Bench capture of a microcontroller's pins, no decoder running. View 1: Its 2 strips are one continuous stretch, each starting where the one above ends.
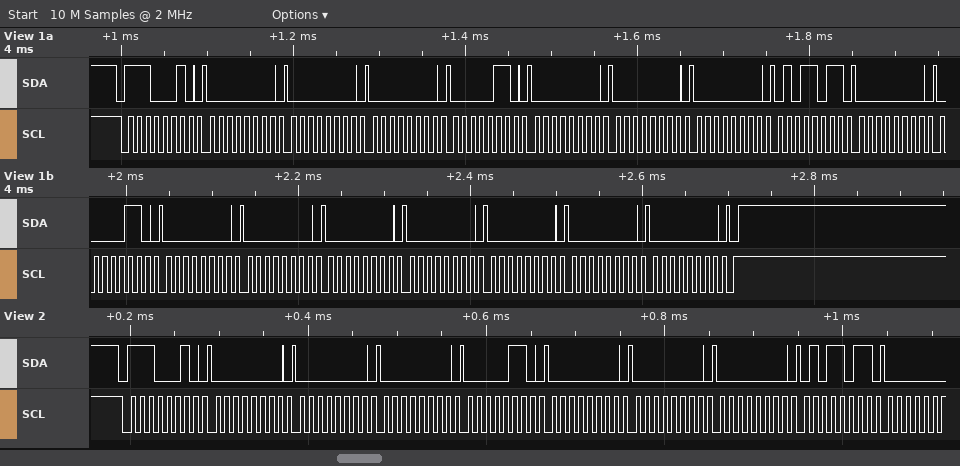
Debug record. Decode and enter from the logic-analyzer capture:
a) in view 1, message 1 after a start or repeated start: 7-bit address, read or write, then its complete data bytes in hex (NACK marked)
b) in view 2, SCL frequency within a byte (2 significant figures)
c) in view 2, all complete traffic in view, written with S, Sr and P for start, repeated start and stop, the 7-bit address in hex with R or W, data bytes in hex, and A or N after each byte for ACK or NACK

0x71 write: 00 00 00 06 00 00 00 5B 00 06 00 00 00 00 00 00 00
100 kHz
S 71W A 00 A 00 A 00 A 06 A 00 A 00 A 00 A 5B A
